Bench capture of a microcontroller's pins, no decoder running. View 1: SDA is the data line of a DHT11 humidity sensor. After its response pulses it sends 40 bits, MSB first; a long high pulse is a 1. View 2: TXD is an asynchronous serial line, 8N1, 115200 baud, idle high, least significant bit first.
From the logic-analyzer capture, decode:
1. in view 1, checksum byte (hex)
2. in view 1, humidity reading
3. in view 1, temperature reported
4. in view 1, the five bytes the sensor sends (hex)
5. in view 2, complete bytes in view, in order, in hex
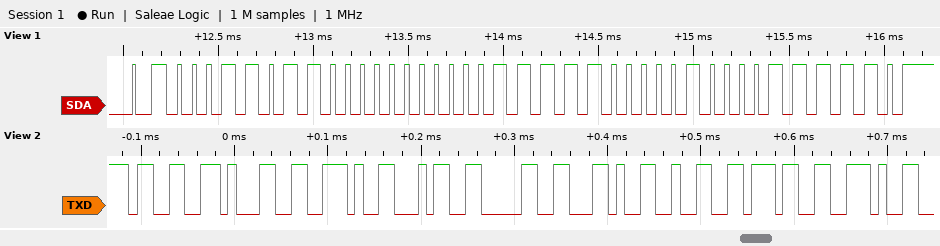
0x3E
27 %
31.4 °C
1B 00 1F 04 3E
0x33 0x31 0x2E 0x34 0x30 0x2C 0x32 0x37 0x2E
